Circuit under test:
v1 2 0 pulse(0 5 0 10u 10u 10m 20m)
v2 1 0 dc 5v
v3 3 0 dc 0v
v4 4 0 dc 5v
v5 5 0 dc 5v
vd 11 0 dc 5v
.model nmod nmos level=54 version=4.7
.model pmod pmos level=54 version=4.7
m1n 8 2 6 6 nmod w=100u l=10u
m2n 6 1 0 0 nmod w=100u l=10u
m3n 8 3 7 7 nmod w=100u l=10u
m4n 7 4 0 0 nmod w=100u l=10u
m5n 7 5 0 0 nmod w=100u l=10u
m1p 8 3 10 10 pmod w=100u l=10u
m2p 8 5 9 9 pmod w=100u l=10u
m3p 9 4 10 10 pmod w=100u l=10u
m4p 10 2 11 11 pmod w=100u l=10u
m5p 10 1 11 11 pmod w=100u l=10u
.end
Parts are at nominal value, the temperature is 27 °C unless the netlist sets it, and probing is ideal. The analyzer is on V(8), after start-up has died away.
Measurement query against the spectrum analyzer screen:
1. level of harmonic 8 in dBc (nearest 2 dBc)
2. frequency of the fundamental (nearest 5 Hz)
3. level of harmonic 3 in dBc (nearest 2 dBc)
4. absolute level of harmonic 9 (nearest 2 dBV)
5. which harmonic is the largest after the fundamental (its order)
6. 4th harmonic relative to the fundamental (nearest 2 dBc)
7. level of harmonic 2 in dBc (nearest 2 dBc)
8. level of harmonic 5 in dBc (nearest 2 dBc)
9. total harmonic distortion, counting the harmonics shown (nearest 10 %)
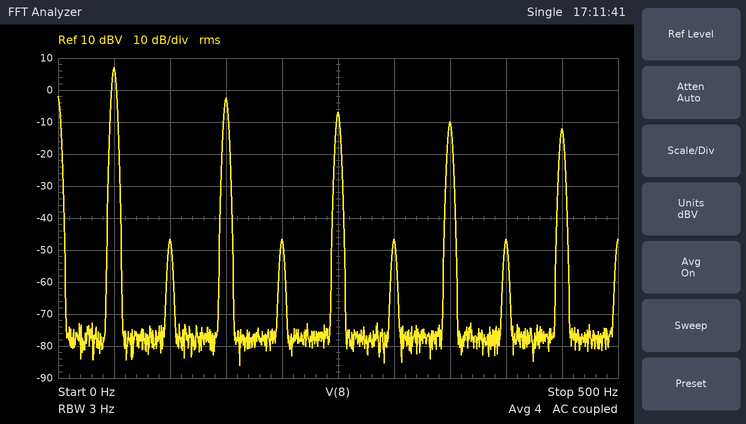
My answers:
-54 dBc
50 Hz
-10 dBc
-12 dBV
3
-54 dBc
-54 dBc
-14 dBc
40 %
